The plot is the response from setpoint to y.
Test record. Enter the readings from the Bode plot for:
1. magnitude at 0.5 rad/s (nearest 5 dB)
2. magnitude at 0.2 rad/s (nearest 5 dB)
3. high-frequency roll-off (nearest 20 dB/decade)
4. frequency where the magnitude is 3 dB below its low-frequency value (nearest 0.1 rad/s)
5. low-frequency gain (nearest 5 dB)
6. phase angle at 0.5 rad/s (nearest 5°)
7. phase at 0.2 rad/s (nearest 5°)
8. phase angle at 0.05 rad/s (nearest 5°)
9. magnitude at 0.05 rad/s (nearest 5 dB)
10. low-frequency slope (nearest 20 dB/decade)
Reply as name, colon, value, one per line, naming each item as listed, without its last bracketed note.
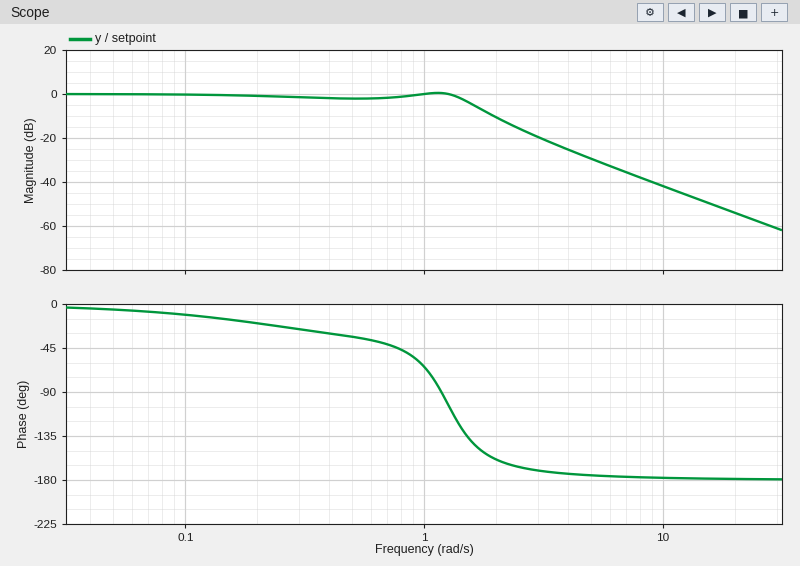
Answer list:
magnitude at 0.5 rad/s: 0 dB
magnitude at 0.2 rad/s: 0 dB
high-frequency roll-off: -40 dB/decade
frequency where the magnitude is 3 dB below its low-frequency value: 1.5 rad/s
low-frequency gain: 0 dB
phase angle at 0.5 rad/s: -35°
phase at 0.2 rad/s: -20°
phase angle at 0.05 rad/s: -5°
magnitude at 0.05 rad/s: 0 dB
low-frequency slope: 0 dB/decade
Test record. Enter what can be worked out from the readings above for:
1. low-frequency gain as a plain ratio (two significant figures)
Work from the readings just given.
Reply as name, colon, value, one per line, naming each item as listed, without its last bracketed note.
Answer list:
low-frequency gain as a plain ratio: 1.0
